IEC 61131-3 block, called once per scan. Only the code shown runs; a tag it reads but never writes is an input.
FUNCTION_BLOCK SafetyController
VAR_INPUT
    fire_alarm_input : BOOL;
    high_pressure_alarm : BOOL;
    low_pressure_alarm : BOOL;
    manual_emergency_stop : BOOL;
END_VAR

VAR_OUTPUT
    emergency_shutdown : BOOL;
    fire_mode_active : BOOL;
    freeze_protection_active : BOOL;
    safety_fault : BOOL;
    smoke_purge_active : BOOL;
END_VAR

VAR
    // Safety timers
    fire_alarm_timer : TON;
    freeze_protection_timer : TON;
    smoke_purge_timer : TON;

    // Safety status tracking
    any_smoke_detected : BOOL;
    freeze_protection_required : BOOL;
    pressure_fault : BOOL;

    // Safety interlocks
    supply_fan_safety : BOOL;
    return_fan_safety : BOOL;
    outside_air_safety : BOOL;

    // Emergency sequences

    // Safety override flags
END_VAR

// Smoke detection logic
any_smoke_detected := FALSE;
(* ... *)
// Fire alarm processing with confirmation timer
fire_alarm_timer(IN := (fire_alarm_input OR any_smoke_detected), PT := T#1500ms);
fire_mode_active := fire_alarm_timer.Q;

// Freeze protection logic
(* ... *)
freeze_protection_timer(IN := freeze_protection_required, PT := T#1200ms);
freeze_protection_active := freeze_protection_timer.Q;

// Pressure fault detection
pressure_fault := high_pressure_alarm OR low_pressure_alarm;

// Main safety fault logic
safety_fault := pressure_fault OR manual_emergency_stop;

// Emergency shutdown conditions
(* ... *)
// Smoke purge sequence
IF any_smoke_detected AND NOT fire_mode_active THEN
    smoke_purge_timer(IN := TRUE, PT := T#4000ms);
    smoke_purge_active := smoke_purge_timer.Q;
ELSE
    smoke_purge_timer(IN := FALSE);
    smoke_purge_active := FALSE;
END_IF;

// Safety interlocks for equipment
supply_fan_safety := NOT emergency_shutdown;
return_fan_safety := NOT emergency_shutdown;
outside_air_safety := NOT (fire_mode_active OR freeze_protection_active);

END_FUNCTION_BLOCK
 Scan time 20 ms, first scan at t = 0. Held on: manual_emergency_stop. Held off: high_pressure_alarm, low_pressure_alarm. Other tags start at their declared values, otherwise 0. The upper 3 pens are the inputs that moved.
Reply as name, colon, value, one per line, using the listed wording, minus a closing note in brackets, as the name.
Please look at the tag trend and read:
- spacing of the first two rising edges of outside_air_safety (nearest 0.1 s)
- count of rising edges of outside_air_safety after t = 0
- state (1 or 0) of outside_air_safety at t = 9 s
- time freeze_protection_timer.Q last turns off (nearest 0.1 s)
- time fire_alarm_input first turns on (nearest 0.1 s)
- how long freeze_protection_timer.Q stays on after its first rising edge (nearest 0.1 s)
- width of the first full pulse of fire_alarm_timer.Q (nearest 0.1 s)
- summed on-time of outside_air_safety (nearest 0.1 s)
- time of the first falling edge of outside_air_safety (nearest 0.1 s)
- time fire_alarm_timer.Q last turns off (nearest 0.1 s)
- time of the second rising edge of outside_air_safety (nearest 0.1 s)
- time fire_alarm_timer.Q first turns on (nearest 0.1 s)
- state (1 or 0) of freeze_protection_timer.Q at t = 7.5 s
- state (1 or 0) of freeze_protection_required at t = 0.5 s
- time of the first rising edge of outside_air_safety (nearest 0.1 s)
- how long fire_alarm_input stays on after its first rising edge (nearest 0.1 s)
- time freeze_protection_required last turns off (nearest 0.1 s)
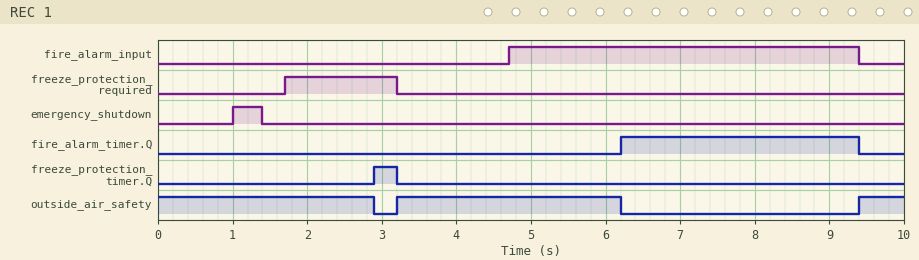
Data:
spacing of the first two rising edges of outside_air_safety: 6.2 s
count of rising edges of outside_air_safety after t = 0: 2
state (1 or 0) of outside_air_safety at t = 9 s: 0
time freeze_protection_timer.Q last turns off: 3.2 s
time fire_alarm_input first turns on: 4.7 s
how long freeze_protection_timer.Q stays on after its first rising edge: 0.3 s
width of the first full pulse of fire_alarm_timer.Q: 3.2 s
summed on-time of outside_air_safety: 6.5 s
time of the first falling edge of outside_air_safety: 2.9 s
time fire_alarm_timer.Q last turns off: 9.4 s
time of the second rising edge of outside_air_safety: 9.4 s
time fire_alarm_timer.Q first turns on: 6.2 s
state (1 or 0) of freeze_protection_timer.Q at t = 7.5 s: 0
state (1 or 0) of freeze_protection_required at t = 0.5 s: 0
time of the first rising edge of outside_air_safety: 3.2 s
how long fire_alarm_input stays on after its first rising edge: 4.7 s
time freeze_protection_required last turns off: 3.2 s
